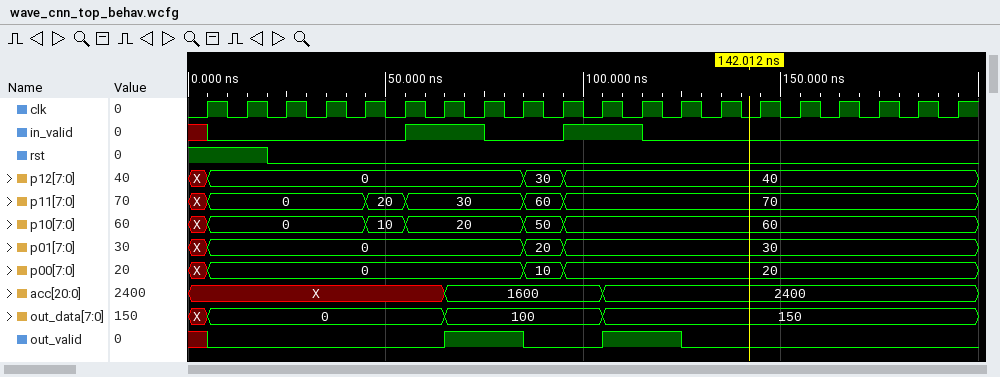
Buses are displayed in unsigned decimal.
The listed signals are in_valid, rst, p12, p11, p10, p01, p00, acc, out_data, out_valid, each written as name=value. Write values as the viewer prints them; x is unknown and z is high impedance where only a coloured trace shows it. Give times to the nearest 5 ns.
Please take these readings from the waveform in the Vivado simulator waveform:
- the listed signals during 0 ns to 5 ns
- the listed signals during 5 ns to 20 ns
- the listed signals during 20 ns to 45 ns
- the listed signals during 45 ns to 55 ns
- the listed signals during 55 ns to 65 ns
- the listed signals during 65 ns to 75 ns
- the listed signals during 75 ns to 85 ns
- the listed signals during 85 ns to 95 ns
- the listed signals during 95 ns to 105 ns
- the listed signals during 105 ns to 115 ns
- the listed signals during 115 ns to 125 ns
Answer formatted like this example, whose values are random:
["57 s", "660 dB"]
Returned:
["in_valid=x, rst=1, p12=X, p11=X, p10=X, p01=X, p00=X, acc=X, out_data=X, out_valid=x", "in_valid=0, rst=1, p12=0, p11=0, p10=0, p01=0, p00=0, acc=X, out_data=0, out_valid=0", "in_valid=0, rst=0, p12=0, p11=0, p10=0, p01=0, p00=0, acc=X, out_data=0, out_valid=0", "in_valid=0, rst=0, p12=0, p11=20, p10=10, p01=0, p00=0, acc=X, out_data=0, out_valid=0", "in_valid=1, rst=0, p12=0, p11=30, p10=20, p01=0, p00=0, acc=X, out_data=0, out_valid=0", "in_valid=1, rst=0, p12=0, p11=30, p10=20, p01=0, p00=0, acc=1600, out_data=100, out_valid=1", "in_valid=0, rst=0, p12=0, p11=30, p10=20, p01=0, p00=0, acc=1600, out_data=100, out_valid=1", "in_valid=0, rst=0, p12=30, p11=60, p10=50, p01=20, p00=10, acc=1600, out_data=100, out_valid=0", "in_valid=1, rst=0, p12=40, p11=70, p10=60, p01=30, p00=20, acc=1600, out_data=100, out_valid=0", "in_valid=1, rst=0, p12=40, p11=70, p10=60, p01=30, p00=20, acc=2400, out_data=150, out_valid=1", "in_valid=0, rst=0, p12=40, p11=70, p10=60, p01=30, p00=20, acc=2400, out_data=150, out_valid=1"]
